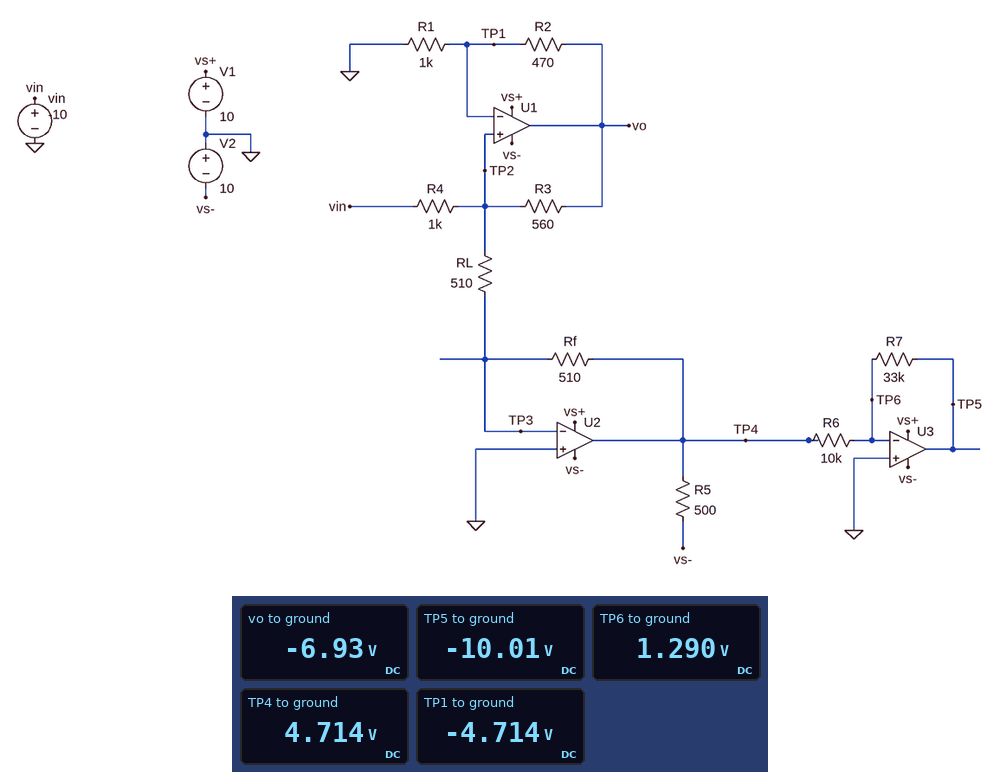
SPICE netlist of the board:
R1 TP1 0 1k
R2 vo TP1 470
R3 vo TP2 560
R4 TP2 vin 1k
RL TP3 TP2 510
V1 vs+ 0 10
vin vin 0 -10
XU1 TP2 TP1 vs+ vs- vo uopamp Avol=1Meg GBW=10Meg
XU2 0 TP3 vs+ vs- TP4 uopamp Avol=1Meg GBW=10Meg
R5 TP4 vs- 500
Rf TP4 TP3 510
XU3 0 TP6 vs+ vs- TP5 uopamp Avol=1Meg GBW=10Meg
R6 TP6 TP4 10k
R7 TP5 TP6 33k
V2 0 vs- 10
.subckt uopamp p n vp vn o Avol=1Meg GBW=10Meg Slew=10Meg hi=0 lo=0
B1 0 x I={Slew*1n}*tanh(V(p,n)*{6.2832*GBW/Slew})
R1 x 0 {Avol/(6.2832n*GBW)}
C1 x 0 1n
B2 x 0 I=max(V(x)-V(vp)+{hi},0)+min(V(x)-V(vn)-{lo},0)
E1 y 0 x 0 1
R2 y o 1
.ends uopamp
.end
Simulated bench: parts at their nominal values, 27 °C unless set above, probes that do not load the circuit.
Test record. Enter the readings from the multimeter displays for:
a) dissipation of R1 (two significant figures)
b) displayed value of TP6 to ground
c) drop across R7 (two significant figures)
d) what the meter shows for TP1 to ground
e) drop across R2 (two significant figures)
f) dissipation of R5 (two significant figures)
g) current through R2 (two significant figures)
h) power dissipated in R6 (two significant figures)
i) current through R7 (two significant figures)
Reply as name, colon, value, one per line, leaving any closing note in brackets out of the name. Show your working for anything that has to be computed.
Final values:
dissipation of R1: (0 V - (-4.714 V))^2 / 1 kΩ = 22 mW
displayed value of TP6 to ground: 1.290 V
drop across R7: 1.29 V - (-10.01 V) = 11 V
what the meter shows for TP1 to ground: -4.714 V
drop across R2: -4.714 V - (-6.93 V) = 2.2 V
dissipation of R5: (4.714 V - (-10 V))^2 / 500 Ω = 430 mW
current through R2: (-4.714 V - (-6.93 V)) / 470 Ω = 4.7 mA
power dissipated in R6: (4.714 V - 1.29 V)^2 / 10 kΩ = 1.2 mW
current through R7: (1.29 V - (-10.01 V)) / 33 kΩ = 340 µA
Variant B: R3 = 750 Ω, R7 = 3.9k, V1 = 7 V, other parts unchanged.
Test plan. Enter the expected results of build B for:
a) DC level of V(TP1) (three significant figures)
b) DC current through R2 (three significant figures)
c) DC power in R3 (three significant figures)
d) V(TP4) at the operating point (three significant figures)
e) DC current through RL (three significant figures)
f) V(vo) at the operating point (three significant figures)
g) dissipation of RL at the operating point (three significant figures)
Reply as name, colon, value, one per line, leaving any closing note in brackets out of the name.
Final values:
DC level of V(TP1): -4.28 V
DC current through R2: 4.28 mA
DC power in R3: 5.41 mW
V(TP4) at the operating point: 4.28 V
DC current through RL: 8.40 mA
V(vo) at the operating point: -6.30 V
dissipation of RL at the operating point: 36.0 mW
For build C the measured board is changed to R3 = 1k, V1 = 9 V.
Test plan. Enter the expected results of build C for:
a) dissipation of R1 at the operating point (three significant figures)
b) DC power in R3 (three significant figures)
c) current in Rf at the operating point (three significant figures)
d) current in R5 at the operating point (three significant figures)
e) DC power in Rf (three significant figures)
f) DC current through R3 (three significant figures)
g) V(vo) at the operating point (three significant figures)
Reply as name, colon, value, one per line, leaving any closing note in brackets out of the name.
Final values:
dissipation of R1 at the operating point: 16.1 mW
DC power in R3: 3.56 mW
current in Rf at the operating point: 7.87 mA
current in R5 at the operating point: 28.0 mA
DC power in Rf: 31.6 mW
DC current through R3: 1.89 mA
V(vo) at the operating point: -5.90 V
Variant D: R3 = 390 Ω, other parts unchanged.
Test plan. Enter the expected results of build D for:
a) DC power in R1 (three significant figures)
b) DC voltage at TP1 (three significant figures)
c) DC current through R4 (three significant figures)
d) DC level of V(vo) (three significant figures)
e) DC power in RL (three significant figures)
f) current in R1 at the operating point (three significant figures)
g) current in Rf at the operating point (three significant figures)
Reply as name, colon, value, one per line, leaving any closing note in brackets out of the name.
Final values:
DC power in R1: 32.4 mW
DC voltage at TP1: -5.70 V
DC current through R4: 4.30 mA
DC level of V(vo): -8.37 V
DC power in RL: 63.6 mW
current in R1 at the operating point: 5.70 mA
current in Rf at the operating point: 11.2 mA
